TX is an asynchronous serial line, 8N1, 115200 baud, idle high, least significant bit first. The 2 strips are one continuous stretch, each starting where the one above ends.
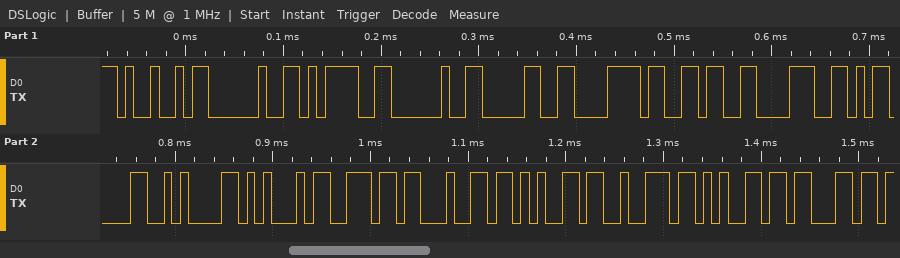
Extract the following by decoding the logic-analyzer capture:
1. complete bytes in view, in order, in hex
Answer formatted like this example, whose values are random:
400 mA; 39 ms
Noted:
0x49 0x20 0x3D 0x20 0x30 0x78 0x36 0x38 0x0D 0x0A 0x45 0x6E 0x64 0x65 0x72 0x65 0x63
